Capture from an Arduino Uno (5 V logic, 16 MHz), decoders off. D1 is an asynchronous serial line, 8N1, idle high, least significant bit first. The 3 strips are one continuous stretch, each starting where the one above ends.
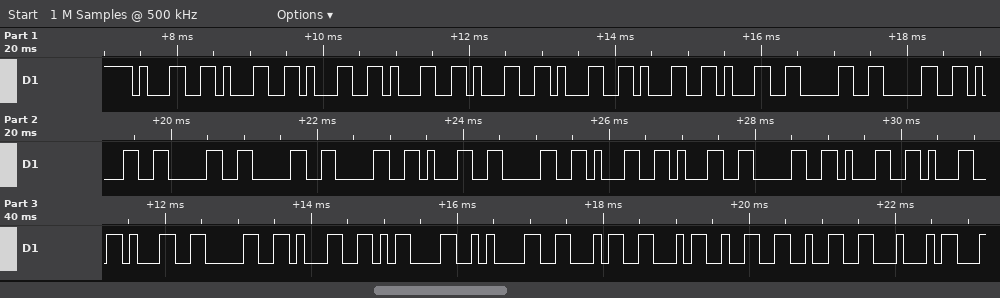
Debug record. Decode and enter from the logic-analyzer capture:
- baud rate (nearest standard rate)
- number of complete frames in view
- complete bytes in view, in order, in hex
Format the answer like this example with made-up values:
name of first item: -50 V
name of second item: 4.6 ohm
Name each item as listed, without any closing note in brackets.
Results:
baud rate: 9600 baud
number of complete frames in view: 31
complete bytes in view, in order, in hex: 0x31 0x31 0x31 0x31 0x31 0x31 0x31 0x31 0x30 0x30 0x31 0x30 0x30 0x30 0x31 0x30 0x31 0x31 0x30 0x31 0x31 0x31 0x30 0x31 0x0D 0x0A 0x46 0x46 0x32 0x32 0x44
